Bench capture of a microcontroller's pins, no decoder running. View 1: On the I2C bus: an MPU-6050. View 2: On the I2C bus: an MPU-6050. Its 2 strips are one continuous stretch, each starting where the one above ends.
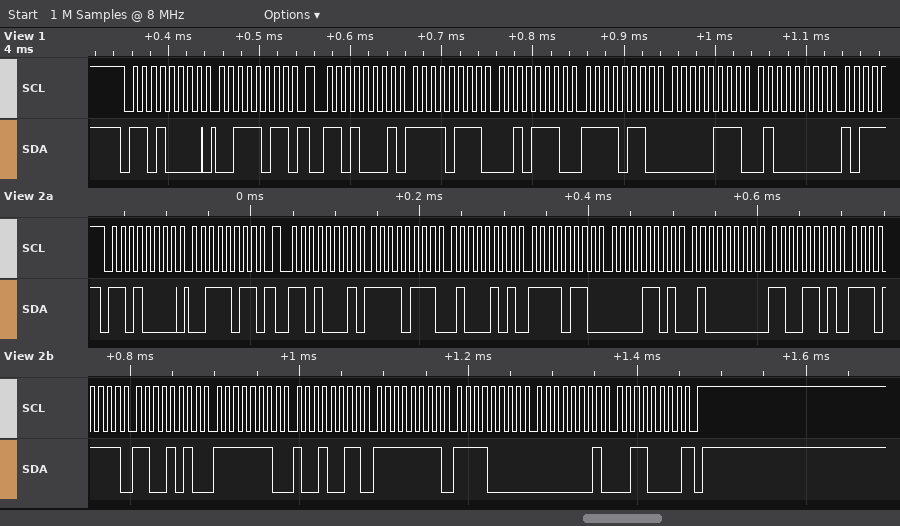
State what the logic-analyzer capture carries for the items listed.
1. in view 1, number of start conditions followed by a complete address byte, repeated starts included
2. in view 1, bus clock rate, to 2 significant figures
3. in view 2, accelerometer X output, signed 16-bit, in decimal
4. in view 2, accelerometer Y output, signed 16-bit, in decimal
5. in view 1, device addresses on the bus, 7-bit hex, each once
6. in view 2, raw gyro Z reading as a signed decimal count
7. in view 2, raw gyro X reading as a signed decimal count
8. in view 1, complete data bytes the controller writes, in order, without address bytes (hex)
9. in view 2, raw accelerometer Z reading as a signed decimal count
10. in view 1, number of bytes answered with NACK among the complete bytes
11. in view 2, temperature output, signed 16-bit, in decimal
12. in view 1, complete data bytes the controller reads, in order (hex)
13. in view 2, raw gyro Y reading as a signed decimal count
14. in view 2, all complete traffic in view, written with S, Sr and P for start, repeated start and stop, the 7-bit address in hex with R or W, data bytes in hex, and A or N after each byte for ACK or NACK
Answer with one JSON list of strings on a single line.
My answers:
["2", "100 kHz", "-2235", "-2547", "0x68", "304", "-365", "3B", "16589", "0", "-4150", "F7 2E F6 07 40", "-16", "S 68W A 3B A Sr 68R A F7 A 45 A F6 A 0D A 40 A CD A EF A CA A FE A 93 A FF A F0 A 01 A 30 N P"]
